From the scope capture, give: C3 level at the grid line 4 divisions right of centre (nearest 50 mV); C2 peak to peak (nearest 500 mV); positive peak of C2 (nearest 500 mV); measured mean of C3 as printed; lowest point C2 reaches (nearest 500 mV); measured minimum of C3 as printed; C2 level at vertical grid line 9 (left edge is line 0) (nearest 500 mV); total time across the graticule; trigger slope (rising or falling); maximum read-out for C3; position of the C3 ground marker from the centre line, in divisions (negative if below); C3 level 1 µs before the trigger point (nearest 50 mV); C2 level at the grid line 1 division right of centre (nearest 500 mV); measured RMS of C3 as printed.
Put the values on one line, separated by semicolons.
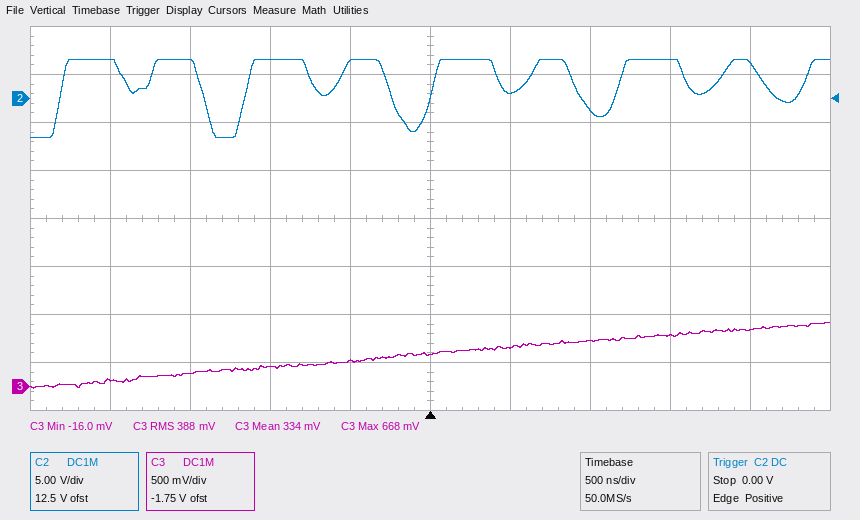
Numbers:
600 mV; 8.0 V; 4.0 V; 334 mV; -4.0 V; -16.0 mV; 3.5 V; 5 µs; rising; 668 mV; -3.5 div; 200 mV; 500 mV; 388 mV
